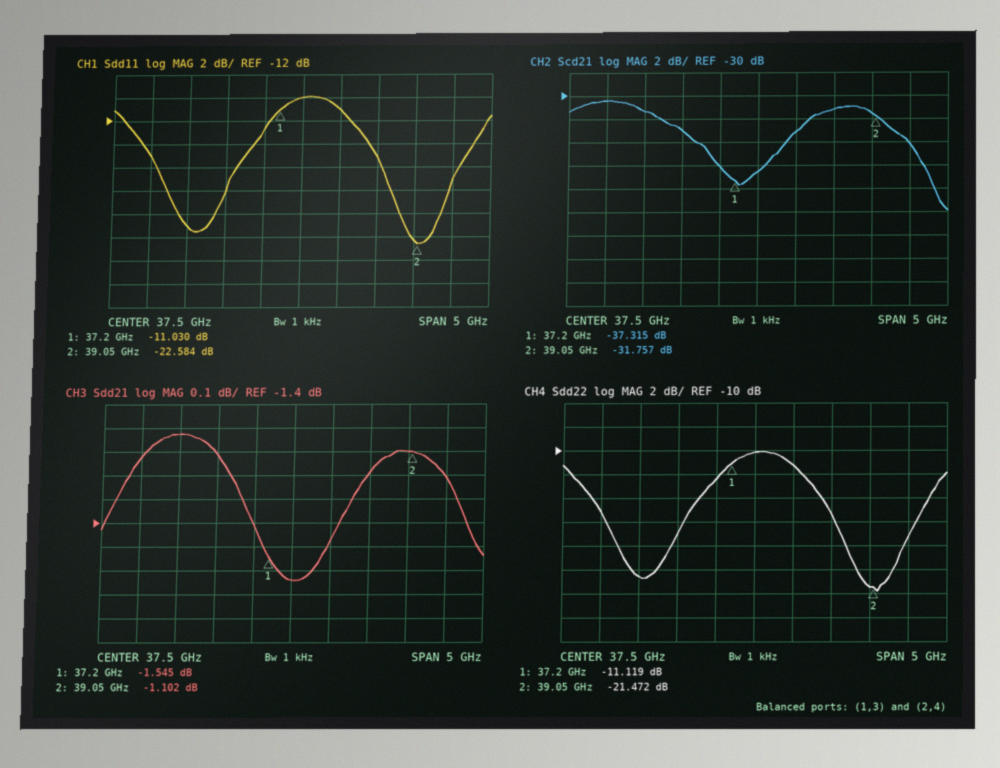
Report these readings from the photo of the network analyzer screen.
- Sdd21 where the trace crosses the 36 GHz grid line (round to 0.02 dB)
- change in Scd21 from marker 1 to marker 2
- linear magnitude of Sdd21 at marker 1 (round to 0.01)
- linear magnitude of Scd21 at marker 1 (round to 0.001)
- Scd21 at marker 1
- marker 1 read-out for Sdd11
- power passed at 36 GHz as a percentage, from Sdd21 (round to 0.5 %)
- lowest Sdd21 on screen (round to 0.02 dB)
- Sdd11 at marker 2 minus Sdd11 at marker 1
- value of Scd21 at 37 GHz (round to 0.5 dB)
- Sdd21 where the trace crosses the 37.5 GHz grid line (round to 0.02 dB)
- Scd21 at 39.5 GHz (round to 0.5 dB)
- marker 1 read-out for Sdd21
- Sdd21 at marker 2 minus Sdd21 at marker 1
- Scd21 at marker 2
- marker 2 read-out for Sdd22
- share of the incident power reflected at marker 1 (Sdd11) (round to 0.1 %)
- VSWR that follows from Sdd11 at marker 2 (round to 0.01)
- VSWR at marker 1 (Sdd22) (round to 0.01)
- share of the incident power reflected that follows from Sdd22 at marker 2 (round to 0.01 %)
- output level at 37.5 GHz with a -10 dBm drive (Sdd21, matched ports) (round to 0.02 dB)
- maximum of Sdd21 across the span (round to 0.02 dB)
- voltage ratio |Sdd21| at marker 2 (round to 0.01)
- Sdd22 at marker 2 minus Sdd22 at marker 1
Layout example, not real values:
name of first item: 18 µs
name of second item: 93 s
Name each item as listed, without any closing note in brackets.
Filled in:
Sdd21 where the trace crosses the 36 GHz grid line: -1.02 dB
change in Scd21 from marker 1 to marker 2: 5.558 dB
linear magnitude of Sdd21 at marker 1: 0.84
linear magnitude of Scd21 at marker 1: 0.014
Scd21 at marker 1: -37.315 dB
marker 1 read-out for Sdd11: -11.030 dB
power passed at 36 GHz as a percentage, from Sdd21: 79.0 %
lowest Sdd21 on screen: -1.64 dB
Sdd11 at marker 2 minus Sdd11 at marker 1: -11.554 dB
value of Scd21 at 37 GHz: -36.0 dB
Sdd21 where the trace crosses the 37.5 GHz grid line: -1.64 dB
Scd21 at 39.5 GHz: -34.0 dB
marker 1 read-out for Sdd21: -1.545 dB
Sdd21 at marker 2 minus Sdd21 at marker 1: 0.443 dB
Scd21 at marker 2: -31.757 dB
marker 2 read-out for Sdd22: -21.472 dB
share of the incident power reflected at marker 1 (Sdd11): 7.9 %
VSWR that follows from Sdd11 at marker 2: 1.16
VSWR at marker 1 (Sdd22): 1.77
share of the incident power reflected that follows from Sdd22 at marker 2: 0.71 %
output level at 37.5 GHz with a -10 dBm drive (Sdd21, matched ports): -11.64 dBm
maximum of Sdd21 across the span: -1.02 dB
voltage ratio |Sdd21| at marker 2: 0.88
Sdd22 at marker 2 minus Sdd22 at marker 1: -10.353 dB
